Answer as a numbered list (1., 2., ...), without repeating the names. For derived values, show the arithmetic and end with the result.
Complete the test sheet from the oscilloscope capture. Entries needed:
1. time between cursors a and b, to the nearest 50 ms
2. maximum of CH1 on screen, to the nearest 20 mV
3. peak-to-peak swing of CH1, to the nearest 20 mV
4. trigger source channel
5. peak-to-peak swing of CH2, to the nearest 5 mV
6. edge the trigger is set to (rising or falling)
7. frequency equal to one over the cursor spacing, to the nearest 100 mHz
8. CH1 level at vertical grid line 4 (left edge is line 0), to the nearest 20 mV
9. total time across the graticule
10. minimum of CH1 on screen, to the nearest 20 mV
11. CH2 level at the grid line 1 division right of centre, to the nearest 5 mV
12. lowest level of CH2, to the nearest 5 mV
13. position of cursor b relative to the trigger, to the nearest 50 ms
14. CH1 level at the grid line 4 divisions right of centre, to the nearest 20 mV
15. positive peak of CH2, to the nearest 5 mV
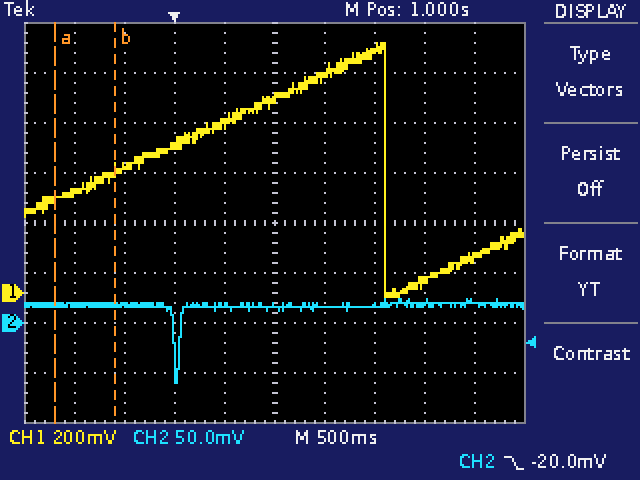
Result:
1. 600 ms
2. 1.00 V
3. 1.00 V − (-20 mV) = 1.02 V
4. CH2
5. 25 mV − (-60 mV) = 85 mV
6. falling
7. 1 / 600 ms ≈ 1.7 Hz
8. 680 mV
9. 5 s
10. -20 mV
11. 15 mV
12. -60 mV
13. -600 ms
14. 140 mV
15. 25 mV
